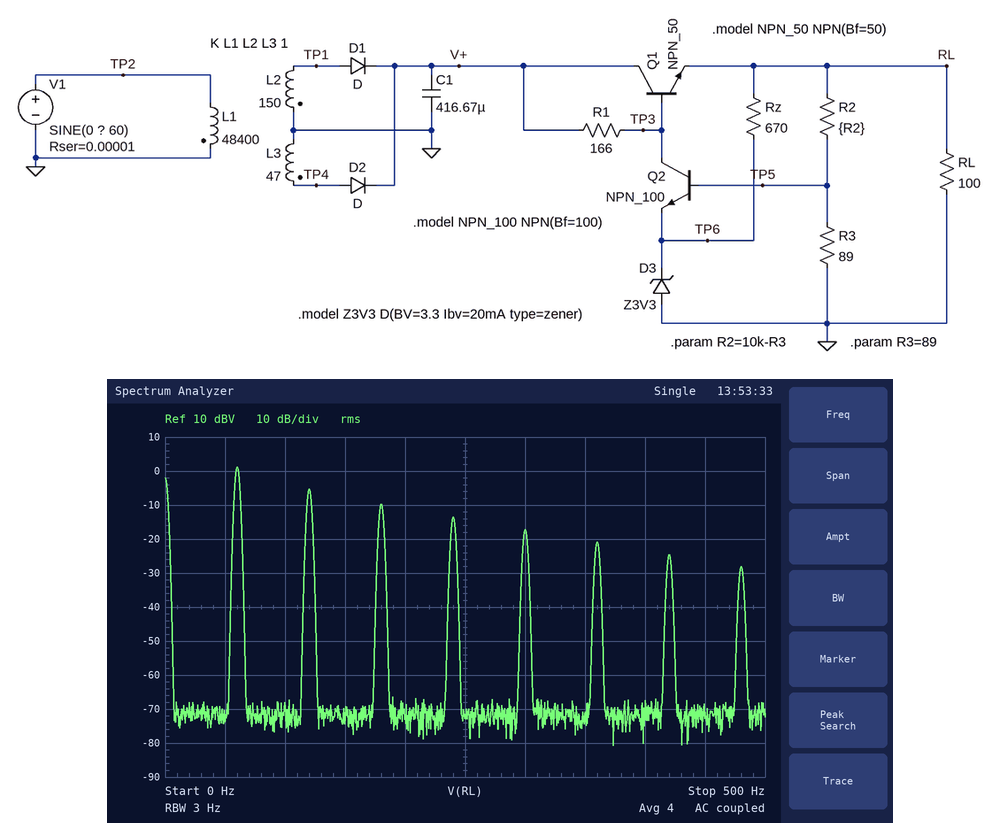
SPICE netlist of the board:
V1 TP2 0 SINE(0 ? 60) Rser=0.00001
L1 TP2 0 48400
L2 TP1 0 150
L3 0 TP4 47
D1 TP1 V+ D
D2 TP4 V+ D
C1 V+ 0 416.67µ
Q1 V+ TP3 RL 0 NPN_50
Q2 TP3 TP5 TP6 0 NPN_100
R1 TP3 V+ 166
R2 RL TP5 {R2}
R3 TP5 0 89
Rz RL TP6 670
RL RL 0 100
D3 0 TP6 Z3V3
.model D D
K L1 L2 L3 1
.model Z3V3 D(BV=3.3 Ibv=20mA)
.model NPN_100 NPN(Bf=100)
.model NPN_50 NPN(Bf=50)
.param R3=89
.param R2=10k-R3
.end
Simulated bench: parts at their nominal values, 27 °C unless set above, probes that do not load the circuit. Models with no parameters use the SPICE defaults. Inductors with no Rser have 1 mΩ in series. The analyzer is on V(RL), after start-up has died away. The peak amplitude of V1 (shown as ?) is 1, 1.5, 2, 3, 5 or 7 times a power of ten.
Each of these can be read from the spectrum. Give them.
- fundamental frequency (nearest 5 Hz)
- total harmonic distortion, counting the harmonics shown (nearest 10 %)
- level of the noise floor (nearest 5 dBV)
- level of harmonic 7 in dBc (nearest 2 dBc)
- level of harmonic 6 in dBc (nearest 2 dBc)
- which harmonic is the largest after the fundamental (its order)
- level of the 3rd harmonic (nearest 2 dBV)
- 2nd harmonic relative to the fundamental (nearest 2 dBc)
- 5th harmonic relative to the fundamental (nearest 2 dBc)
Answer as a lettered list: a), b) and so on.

a) 60 Hz
b) 60 %
c) -70 dBV
d) -26 dBc
e) -22 dBc
f) 2
g) -10 dBV
h) -6 dBc
i) -18 dBc
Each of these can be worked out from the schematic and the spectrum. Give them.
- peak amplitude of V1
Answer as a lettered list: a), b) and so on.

a) 300 V
